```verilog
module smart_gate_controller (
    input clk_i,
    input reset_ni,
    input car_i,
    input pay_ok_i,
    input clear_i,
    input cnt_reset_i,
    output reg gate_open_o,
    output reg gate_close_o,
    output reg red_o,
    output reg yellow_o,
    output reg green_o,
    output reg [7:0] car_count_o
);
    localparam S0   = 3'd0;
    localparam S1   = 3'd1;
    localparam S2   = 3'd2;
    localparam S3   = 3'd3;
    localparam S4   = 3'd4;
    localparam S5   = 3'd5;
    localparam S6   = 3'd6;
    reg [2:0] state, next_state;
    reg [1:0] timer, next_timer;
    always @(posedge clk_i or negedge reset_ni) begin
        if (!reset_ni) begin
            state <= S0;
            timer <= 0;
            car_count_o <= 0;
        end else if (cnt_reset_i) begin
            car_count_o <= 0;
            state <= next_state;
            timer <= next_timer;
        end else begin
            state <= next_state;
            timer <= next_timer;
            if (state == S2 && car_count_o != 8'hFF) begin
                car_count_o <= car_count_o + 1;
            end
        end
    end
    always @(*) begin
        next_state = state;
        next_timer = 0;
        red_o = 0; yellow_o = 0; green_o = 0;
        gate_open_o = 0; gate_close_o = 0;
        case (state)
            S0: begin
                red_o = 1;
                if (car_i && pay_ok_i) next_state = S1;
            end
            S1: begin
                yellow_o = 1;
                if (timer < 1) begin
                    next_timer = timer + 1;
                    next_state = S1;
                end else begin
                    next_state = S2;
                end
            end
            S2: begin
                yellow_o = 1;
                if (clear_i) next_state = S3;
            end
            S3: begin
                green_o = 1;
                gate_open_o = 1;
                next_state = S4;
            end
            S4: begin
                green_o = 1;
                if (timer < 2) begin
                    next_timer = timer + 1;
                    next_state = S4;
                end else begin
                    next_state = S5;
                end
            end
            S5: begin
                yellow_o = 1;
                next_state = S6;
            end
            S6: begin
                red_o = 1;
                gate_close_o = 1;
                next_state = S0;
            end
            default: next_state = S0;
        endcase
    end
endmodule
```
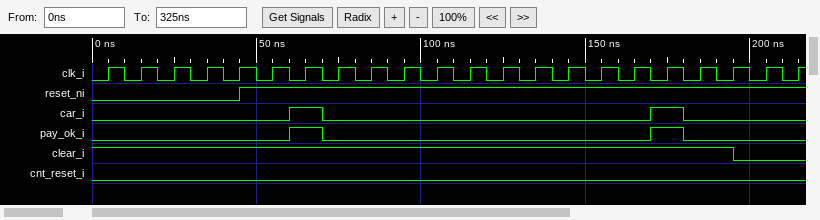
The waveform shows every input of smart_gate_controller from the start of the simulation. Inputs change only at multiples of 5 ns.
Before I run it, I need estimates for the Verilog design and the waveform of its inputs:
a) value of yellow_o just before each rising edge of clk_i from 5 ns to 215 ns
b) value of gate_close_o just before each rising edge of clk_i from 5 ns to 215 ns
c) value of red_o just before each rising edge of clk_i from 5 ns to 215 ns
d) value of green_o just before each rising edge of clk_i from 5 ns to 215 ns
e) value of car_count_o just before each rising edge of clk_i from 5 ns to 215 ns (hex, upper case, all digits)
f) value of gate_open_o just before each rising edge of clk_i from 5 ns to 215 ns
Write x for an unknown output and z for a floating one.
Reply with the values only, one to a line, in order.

0 0 0 0 0 0 0 1 1 1 0 0 0 0 1 0 0 0 1 1 1 1
0 0 0 0 0 0 0 0 0 0 0 0 0 0 0 1 0 0 0 0 0 0
1 1 1 1 1 1 1 0 0 0 0 0 0 0 0 1 1 1 0 0 0 0
0 0 0 0 0 0 0 0 0 0 1 1 1 1 0 0 0 0 0 0 0 0
00, 00, 00, 00, 00, 00, 00, 00, 00, 00, 01, 01, 01, 01, 01, 01, 01, 01, 01, 01, 01, 02
0 0 0 0 0 0 0 0 0 0 1 0 0 0 0 0 0 0 0 0 0 0
